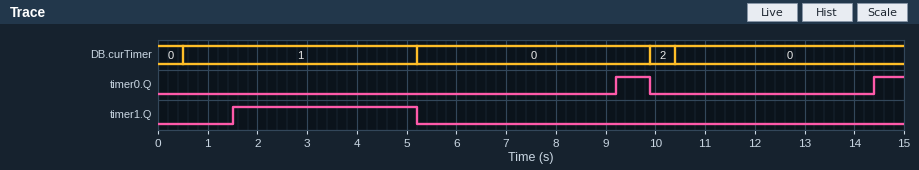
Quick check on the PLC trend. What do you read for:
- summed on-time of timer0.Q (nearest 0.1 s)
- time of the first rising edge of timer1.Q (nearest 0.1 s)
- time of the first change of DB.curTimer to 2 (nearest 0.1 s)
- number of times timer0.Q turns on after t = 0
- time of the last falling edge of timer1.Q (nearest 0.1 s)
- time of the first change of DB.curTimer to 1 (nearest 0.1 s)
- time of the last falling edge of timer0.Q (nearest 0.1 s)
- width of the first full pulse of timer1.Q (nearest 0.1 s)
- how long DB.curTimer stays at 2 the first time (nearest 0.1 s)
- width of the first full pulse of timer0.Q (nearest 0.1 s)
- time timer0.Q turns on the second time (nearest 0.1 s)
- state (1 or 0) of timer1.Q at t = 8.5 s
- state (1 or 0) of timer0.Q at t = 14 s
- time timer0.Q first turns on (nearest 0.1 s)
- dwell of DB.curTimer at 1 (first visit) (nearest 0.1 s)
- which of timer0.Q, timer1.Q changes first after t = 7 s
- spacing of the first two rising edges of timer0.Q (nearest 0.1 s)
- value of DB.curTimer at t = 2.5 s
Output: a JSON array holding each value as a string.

["1.3 s", "1.5 s", "9.9 s", "2", "5.2 s", "0.5 s", "9.9 s", "3.7 s", "0.5 s", "0.7 s", "14.4 s", "0", "0", "9.2 s", "4.7 s", "timer0.Q", "5.2 s", "1"]
